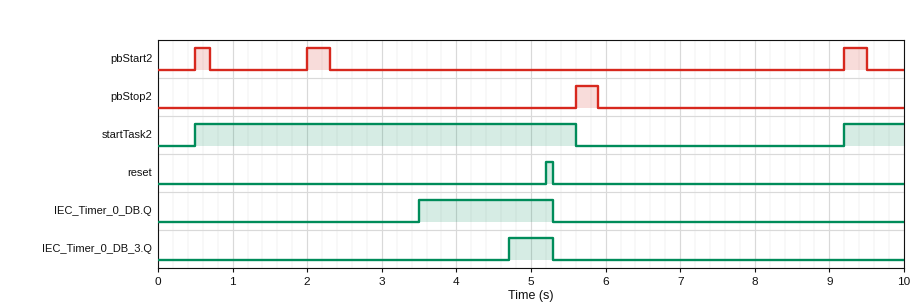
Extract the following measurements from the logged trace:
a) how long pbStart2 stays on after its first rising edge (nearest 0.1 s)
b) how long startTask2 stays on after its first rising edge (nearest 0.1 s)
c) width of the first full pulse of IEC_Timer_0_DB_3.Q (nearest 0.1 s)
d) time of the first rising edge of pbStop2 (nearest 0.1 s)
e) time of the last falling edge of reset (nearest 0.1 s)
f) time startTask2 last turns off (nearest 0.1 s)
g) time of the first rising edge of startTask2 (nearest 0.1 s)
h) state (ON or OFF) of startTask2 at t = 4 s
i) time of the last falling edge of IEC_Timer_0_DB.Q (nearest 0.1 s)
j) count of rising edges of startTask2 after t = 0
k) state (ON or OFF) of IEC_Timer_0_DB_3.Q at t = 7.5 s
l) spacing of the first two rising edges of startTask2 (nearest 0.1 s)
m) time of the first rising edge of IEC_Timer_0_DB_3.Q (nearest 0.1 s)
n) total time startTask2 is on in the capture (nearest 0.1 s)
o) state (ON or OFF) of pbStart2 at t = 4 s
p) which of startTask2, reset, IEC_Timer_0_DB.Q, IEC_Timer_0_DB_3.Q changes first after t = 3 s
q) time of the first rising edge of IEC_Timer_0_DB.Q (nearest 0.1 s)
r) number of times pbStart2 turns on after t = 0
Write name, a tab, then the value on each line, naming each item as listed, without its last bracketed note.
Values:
how long pbStart2 stays on after its first rising edge	0.2 s
how long startTask2 stays on after its first rising edge	5.1 s
width of the first full pulse of IEC_Timer_0_DB_3.Q	0.6 s
time of the first rising edge of pbStop2	5.6 s
time of the last falling edge of reset	5.3 s
time startTask2 last turns off	5.6 s
time of the first rising edge of startTask2	0.5 s
state (ON or OFF) of startTask2 at t = 4 s	ON
time of the last falling edge of IEC_Timer_0_DB.Q	5.3 s
count of rising edges of startTask2 after t = 0	2
state (ON or OFF) of IEC_Timer_0_DB_3.Q at t = 7.5 s	OFF
spacing of the first two rising edges of startTask2	8.7 s
time of the first rising edge of IEC_Timer_0_DB_3.Q	4.7 s
total time startTask2 is on in the capture	5.9 s
state (ON or OFF) of pbStart2 at t = 4 s	OFF
which of startTask2, reset, IEC_Timer_0_DB.Q, IEC_Timer_0_DB_3.Q changes first after t = 3 s	IEC_Timer_0_DB.Q
time of the first rising edge of IEC_Timer_0_DB.Q	3.5 s
number of times pbStart2 turns on after t = 0	3
